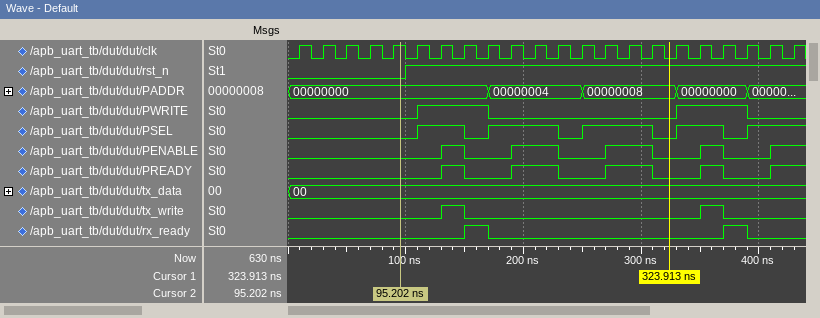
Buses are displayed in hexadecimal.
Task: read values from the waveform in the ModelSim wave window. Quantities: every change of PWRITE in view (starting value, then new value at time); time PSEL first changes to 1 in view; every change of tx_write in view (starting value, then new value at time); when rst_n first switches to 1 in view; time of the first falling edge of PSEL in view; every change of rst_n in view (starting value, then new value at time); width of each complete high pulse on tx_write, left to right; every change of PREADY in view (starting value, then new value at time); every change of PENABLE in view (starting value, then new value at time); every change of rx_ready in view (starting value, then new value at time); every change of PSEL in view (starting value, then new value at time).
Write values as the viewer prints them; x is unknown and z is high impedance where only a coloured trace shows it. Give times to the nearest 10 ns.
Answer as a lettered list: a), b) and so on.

a) 0, 1 at 110 ns, 0 at 170 ns, 1 at 330 ns, 0 at 390 ns
b) 110 ns
c) 0, 1 at 130 ns, 0 at 150 ns, 1 at 350 ns, 0 at 370 ns
d) 100 ns
e) 150 ns
f) 0, 1 at 100 ns
g) 20 ns, 20 ns
h) 0, 1 at 130 ns, 0 at 150 ns, 1 at 190 ns, 0 at 230 ns, 1 at 270 ns, 0 at 310 ns, 1 at 350 ns, 0 at 370 ns, 1 at 410 ns
i) 0, 1 at 130 ns, 0 at 150 ns, 1 at 190 ns, 0 at 230 ns, 1 at 270 ns, 0 at 310 ns, 1 at 350 ns, 0 at 370 ns, 1 at 410 ns
j) 0, 1 at 150 ns, 0 at 170 ns, 1 at 370 ns, 0 at 390 ns
k) 0, 1 at 110 ns, 0 at 150 ns, 1 at 170 ns, 0 at 230 ns, 1 at 250 ns, 0 at 310 ns, 1 at 330 ns, 0 at 370 ns, 1 at 390 ns
